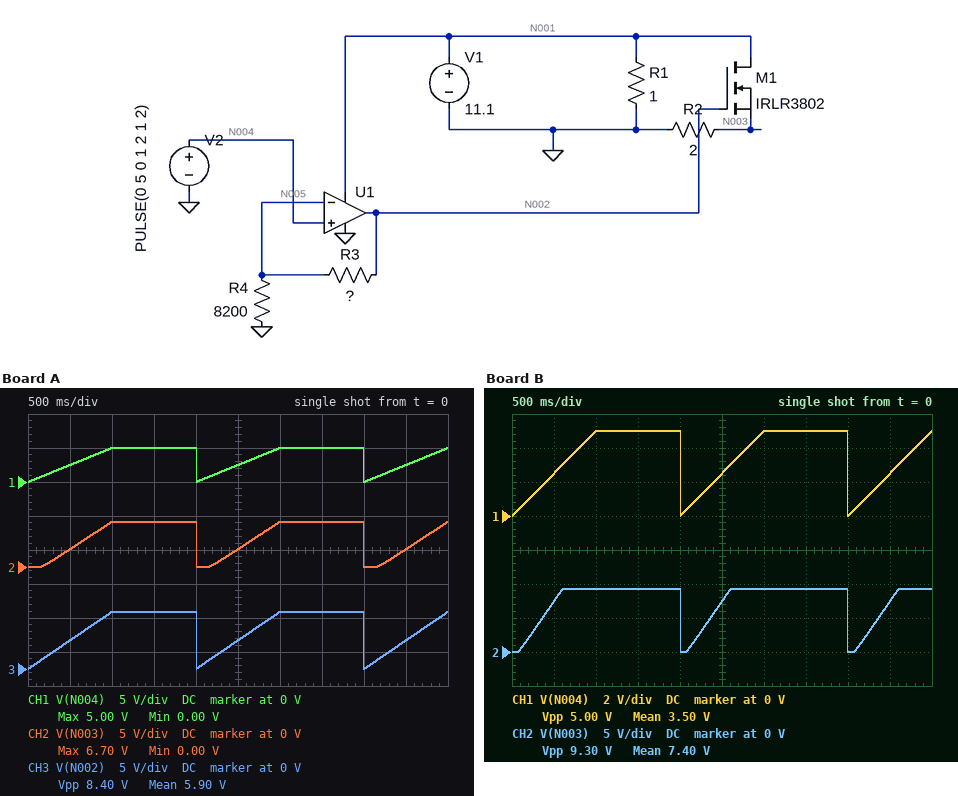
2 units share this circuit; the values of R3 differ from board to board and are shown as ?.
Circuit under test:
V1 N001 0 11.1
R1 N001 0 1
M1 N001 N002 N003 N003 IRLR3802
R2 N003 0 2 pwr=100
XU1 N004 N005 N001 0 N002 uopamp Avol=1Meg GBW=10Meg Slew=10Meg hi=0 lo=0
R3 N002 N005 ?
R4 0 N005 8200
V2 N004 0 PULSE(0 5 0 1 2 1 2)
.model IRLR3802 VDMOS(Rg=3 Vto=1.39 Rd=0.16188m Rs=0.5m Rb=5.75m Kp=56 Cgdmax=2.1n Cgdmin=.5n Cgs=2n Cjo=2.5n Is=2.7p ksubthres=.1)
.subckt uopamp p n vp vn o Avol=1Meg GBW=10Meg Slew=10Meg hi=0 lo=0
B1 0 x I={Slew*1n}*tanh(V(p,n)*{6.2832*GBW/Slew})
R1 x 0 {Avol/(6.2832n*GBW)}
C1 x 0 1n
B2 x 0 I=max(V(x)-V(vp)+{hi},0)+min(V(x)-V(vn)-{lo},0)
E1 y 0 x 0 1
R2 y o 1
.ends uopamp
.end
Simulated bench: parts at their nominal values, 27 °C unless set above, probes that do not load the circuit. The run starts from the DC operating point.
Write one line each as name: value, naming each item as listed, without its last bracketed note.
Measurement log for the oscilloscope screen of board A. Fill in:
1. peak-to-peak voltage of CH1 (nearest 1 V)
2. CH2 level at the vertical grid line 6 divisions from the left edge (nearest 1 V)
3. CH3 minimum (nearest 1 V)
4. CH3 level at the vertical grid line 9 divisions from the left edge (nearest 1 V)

peak-to-peak voltage of CH1: 5 V
CH2 level at the vertical grid line 6 divisions from the left edge: 7 V
CH3 minimum: 0 V
CH3 level at the vertical grid line 9 divisions from the left edge: 4 V
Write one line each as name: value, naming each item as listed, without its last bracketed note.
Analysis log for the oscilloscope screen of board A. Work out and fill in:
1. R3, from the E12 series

R3, from the E12 series: 5.6 kΩ
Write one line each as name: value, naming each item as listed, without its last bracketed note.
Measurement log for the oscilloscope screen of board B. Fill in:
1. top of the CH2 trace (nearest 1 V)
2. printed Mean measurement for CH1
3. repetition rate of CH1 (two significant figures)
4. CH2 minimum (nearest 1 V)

top of the CH2 trace: 9 V
printed Mean measurement for CH1: 3.50 V
repetition rate of CH1: 500 mHz
CH2 minimum: 0 V
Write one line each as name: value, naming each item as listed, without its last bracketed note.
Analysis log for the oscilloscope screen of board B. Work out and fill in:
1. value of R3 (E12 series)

value of R3: 22 kΩ
